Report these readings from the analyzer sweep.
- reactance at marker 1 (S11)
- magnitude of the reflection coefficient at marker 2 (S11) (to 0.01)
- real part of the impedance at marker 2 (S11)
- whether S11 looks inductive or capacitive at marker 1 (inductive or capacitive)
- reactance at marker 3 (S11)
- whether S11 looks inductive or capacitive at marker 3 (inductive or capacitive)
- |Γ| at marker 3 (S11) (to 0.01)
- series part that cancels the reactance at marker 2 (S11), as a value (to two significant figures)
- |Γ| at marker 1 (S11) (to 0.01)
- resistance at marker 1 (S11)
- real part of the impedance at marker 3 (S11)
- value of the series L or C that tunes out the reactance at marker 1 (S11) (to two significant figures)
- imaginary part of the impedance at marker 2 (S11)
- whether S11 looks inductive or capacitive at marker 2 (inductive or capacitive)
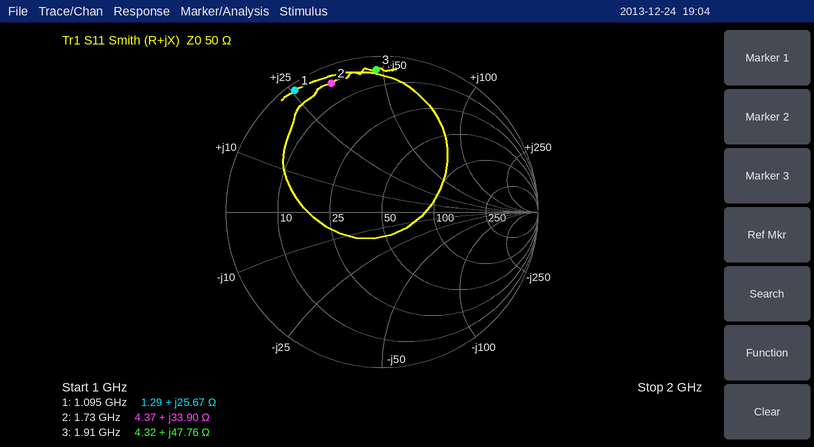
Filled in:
+25.67 Ω
0.89
4.37 Ω
inductive
+47.76 Ω
inductive
0.91
2.7 pF
0.96
1.29 Ω
4.32 Ω
5.7 pF
+33.90 Ω
inductive
